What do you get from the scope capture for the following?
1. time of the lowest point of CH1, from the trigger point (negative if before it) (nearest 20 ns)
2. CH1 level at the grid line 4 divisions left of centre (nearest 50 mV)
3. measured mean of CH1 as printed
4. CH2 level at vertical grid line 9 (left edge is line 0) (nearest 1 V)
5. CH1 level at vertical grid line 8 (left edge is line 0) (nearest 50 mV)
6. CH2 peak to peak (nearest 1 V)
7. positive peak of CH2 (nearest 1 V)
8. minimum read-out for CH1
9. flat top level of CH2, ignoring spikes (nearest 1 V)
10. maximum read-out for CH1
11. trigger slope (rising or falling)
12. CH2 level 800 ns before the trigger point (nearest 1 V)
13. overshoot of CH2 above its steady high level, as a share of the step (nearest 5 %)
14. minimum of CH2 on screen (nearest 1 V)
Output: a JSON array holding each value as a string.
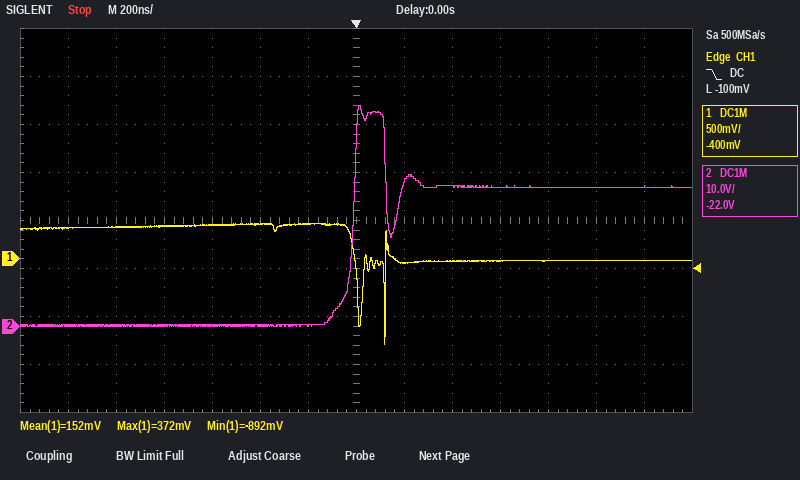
["+120 ns", "350 mV", "152 mV", "29 V", "-50 mV", "46 V", "46 V", "-892 mV", "29 V", "372 mV", "falling", "0 V", "60 %", "0 V"]
